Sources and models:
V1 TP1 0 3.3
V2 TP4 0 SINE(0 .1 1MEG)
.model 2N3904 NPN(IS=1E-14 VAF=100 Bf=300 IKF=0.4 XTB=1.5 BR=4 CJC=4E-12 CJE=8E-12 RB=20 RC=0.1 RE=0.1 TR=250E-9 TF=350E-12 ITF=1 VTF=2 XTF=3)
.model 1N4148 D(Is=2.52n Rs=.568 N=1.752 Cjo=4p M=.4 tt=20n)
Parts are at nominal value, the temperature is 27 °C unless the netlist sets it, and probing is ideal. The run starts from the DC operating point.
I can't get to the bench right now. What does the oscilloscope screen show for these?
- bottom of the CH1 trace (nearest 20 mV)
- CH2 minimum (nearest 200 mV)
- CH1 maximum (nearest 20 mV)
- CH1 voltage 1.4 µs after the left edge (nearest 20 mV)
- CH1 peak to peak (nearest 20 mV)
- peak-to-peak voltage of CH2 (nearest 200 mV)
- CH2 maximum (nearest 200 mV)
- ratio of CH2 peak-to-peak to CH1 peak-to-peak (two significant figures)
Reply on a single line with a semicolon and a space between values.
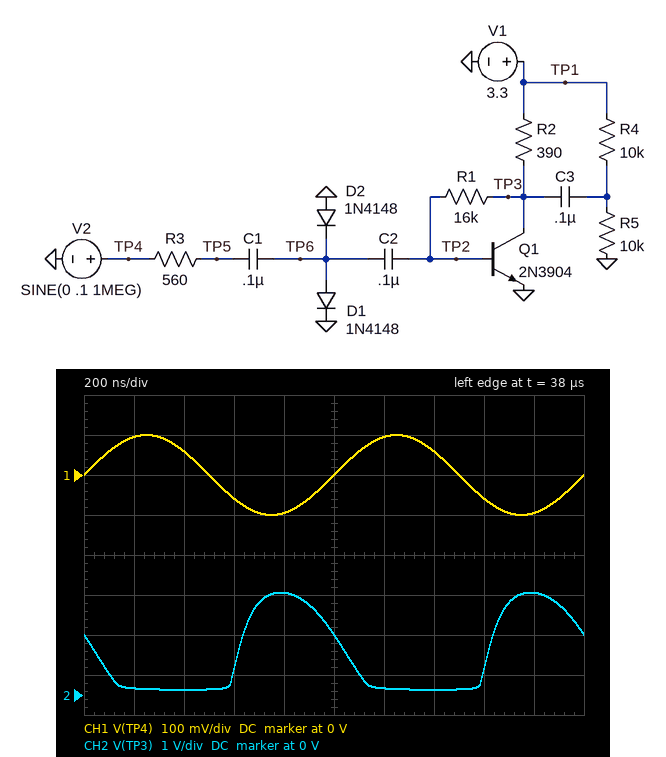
-100 mV; 200 mV; 100 mV; 60 mV; 200 mV; 2.4 V; 2.6 V; 12
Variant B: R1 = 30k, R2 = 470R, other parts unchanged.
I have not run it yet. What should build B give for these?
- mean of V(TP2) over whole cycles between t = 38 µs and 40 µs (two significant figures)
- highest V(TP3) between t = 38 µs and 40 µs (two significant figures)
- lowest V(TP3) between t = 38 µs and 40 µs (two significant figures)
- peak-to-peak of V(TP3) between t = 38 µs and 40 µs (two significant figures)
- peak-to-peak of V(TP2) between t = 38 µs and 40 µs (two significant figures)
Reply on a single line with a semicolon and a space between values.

690 mV; 2.9 V; 120 mV; 2.8 V; 76 mV
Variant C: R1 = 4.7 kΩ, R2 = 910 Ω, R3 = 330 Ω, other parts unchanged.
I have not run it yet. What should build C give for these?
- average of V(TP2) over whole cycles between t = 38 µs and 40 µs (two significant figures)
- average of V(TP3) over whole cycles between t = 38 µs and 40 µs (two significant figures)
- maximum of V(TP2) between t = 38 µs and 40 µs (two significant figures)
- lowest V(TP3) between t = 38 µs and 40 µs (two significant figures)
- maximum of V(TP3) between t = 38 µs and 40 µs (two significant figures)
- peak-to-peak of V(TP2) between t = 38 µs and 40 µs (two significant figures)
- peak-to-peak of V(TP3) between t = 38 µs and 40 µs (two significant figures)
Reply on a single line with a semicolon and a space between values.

680 mV; 750 mV; 690 mV; 99 mV; 1.8 V; 34 mV; 1.7 V
